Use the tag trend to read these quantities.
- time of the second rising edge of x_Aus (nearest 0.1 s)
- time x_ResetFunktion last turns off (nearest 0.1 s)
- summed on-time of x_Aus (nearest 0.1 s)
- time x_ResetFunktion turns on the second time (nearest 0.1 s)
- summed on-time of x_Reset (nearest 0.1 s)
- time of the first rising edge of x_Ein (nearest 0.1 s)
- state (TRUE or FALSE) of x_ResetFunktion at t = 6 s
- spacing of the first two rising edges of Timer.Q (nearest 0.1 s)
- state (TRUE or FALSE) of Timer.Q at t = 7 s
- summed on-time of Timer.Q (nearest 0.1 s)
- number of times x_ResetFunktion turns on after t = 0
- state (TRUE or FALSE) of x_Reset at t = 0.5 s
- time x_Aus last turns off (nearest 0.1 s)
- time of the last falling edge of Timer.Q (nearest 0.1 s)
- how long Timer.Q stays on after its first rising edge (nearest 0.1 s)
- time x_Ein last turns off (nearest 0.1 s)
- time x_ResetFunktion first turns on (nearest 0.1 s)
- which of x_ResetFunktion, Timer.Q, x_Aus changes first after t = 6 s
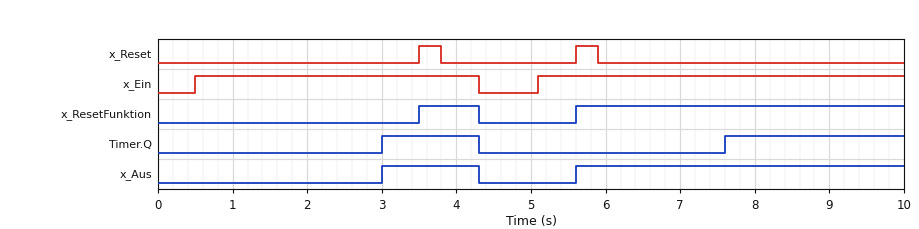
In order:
5.6 s
4.3 s
5.7 s
5.6 s
0.6 s
0.5 s
TRUE
4.6 s
FALSE
3.7 s
2
FALSE
4.3 s
4.3 s
1.3 s
4.3 s
3.5 s
Timer.Q
